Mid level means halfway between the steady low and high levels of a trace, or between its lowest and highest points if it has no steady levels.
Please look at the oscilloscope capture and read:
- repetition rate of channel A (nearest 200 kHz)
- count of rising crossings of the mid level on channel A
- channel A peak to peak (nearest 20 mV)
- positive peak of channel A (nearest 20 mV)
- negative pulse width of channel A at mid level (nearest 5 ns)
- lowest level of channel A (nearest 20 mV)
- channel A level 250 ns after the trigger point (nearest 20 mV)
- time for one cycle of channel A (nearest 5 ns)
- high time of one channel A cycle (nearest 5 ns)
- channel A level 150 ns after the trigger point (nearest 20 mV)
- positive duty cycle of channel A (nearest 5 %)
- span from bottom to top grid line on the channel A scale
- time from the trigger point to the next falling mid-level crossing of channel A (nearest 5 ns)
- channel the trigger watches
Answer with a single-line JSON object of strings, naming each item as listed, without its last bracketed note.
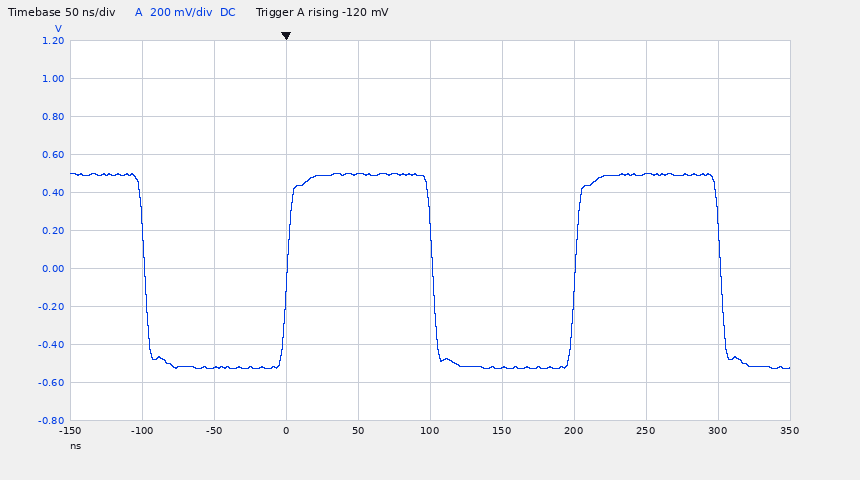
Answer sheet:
{"repetition rate of channel A": "5.0 MHz", "count of rising crossings of the mid level on channel A": "2", "channel A peak to peak": "1.02 V", "positive peak of channel A": "500 mV", "negative pulse width of channel A at mid level": "100 ns", "lowest level of channel A": "-520 mV", "channel A level 250 ns after the trigger point": "500 mV", "time for one cycle of channel A": "200 ns", "high time of one channel A cycle": "100 ns", "channel A level 150 ns after the trigger point": "-520 mV", "positive duty cycle of channel A": "50 %", "span from bottom to top grid line on the channel A scale": "2 V", "time from the trigger point to the next falling mid-level crossing of channel A": "100 ns", "channel the trigger watches": "channel A"}
